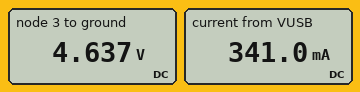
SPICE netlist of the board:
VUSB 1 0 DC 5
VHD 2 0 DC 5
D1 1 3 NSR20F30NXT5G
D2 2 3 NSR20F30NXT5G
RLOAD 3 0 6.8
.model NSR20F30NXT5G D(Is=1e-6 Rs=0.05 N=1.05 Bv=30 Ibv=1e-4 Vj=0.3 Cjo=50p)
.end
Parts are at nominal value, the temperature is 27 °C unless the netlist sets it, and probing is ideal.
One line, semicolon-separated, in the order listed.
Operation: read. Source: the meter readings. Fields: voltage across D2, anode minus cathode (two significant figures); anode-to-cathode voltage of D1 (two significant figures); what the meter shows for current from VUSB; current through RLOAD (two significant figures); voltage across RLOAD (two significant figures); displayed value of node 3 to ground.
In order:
360 mV; 360 mV; 341.0 mA; 680 mA; 4.6 V; 4.637 V
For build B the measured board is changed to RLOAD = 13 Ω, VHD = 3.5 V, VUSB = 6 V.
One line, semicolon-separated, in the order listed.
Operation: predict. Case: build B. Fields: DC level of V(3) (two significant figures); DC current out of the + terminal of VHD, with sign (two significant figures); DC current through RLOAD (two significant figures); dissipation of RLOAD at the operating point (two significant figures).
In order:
5.6 V; -1.0 µA; 430 mA; 2.4 W
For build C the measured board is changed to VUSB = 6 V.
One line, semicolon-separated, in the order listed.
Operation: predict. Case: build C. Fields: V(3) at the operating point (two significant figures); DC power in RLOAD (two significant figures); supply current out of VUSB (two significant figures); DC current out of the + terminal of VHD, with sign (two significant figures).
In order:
5.6 V; 4.6 W; 820 mA; -1.0 µA
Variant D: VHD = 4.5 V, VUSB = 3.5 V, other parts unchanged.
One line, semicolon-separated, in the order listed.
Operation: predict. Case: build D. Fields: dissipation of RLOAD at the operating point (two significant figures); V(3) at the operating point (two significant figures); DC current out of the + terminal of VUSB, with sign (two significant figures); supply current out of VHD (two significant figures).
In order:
2.5 W; 4.1 V; -1.0 µA; 600 mA
